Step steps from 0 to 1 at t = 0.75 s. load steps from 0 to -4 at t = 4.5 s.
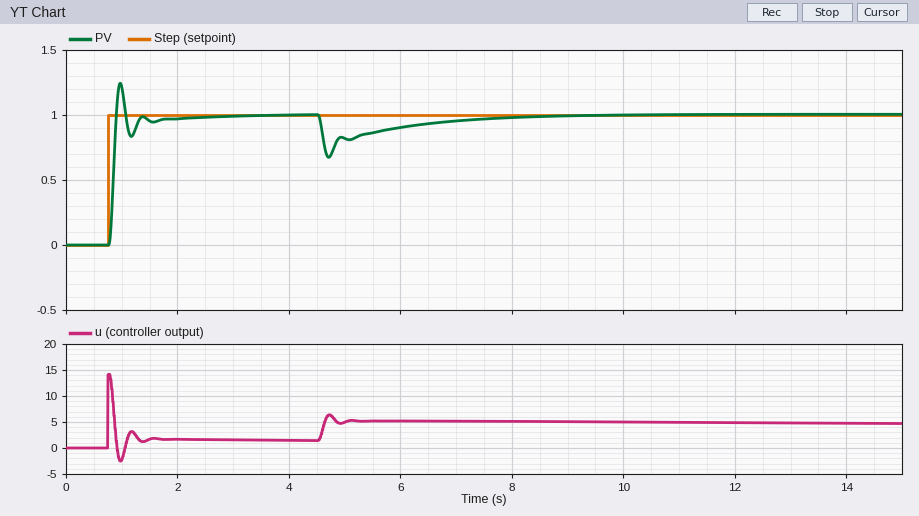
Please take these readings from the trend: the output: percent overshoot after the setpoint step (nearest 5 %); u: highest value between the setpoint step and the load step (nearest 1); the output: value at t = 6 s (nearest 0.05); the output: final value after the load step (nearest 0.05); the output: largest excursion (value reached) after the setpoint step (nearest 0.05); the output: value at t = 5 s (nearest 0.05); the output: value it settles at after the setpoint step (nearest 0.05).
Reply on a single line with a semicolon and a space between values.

25 %; 14; 0.90; 1.00; 1.25; 0.80; 1.00
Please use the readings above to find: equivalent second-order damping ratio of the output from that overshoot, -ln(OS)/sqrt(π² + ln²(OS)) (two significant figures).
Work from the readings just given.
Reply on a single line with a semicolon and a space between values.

0.40
